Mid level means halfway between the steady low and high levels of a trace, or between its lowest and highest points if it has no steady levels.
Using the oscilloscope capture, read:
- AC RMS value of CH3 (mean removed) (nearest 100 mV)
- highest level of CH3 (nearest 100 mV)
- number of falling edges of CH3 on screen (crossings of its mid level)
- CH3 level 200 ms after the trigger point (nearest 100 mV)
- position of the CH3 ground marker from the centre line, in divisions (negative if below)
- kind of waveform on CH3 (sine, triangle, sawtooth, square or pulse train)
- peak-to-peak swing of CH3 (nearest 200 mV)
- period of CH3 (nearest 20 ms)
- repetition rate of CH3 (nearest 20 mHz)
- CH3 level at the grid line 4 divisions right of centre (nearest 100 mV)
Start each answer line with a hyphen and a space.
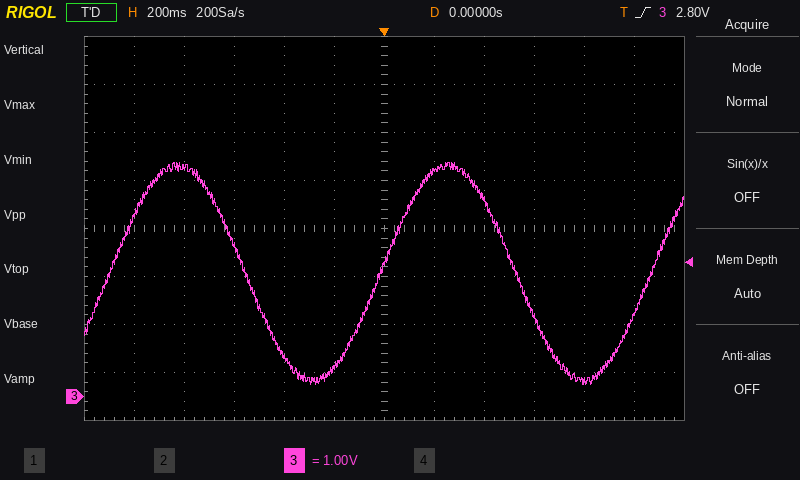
- 1.6 V
- 4.9 V
- 2
- 4.7 V
- -3.5 div
- sine
- 4.6 V
- 1.08 s
- 920 mHz
- 300 mV
